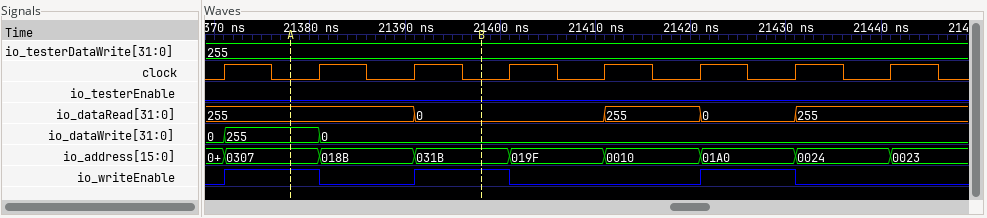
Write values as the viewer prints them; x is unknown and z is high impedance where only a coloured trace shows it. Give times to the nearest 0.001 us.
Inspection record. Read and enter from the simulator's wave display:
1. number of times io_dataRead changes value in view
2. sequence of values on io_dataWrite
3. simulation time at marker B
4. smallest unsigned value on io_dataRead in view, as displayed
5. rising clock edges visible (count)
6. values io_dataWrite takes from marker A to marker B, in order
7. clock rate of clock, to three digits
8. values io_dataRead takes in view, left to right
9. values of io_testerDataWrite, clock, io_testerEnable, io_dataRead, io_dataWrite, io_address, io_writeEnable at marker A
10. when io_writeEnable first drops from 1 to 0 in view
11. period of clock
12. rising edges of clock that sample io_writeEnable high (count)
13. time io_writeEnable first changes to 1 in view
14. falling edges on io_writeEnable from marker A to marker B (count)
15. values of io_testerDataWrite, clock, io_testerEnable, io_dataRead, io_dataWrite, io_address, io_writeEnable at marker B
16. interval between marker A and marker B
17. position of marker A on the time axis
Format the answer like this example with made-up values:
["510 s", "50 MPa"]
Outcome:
["4", "0, 255, 0", "21.398 us", "0", "8", "255, 0", "100 MHz", "255, 0, 255, 0, 255", "io_testerDataWrite=255, clock=0, io_testerEnable=0, io_dataRead=255, io_dataWrite=255, io_address=0307, io_writeEnable=1", "21.381 us", "0.01 us", "3", "21.371 us", "1", "io_testerDataWrite=255, clock=0, io_testerEnable=0, io_dataRead=0, io_dataWrite=0, io_address=031B, io_writeEnable=1", "0.02 us", "21.378 us"]
